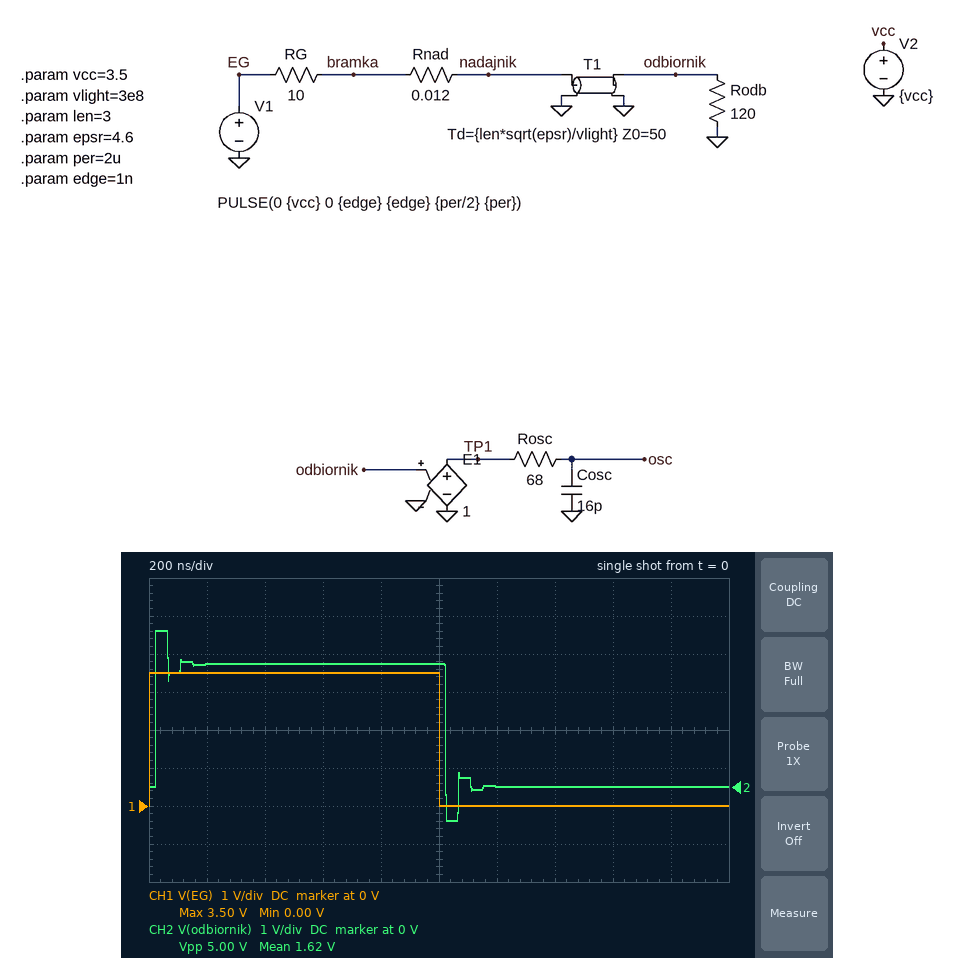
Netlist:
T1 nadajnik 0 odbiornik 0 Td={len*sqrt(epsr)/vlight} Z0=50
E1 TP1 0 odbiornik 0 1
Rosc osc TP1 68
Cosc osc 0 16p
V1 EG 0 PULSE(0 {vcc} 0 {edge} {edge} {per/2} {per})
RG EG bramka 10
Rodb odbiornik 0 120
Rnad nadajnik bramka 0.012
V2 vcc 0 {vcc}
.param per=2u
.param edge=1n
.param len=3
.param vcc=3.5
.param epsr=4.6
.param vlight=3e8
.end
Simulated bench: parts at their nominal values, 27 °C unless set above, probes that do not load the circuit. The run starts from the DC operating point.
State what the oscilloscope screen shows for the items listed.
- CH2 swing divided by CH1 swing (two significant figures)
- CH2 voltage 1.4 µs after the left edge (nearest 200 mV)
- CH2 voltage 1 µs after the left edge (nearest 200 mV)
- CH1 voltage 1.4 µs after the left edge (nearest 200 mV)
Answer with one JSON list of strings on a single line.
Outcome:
["1.4", "0 V", "3.2 V", "0 V"]
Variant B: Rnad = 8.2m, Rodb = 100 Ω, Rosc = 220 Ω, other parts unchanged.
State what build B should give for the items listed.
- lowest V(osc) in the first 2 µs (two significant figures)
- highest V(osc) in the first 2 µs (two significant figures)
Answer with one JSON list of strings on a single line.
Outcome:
["-710 mV", "3.9 V"]
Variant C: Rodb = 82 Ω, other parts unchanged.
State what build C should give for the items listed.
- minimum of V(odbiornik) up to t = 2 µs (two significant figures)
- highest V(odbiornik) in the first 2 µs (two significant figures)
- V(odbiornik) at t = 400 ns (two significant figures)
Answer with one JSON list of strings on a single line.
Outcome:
["-500 mV", "3.6 V", "3.1 V"]
